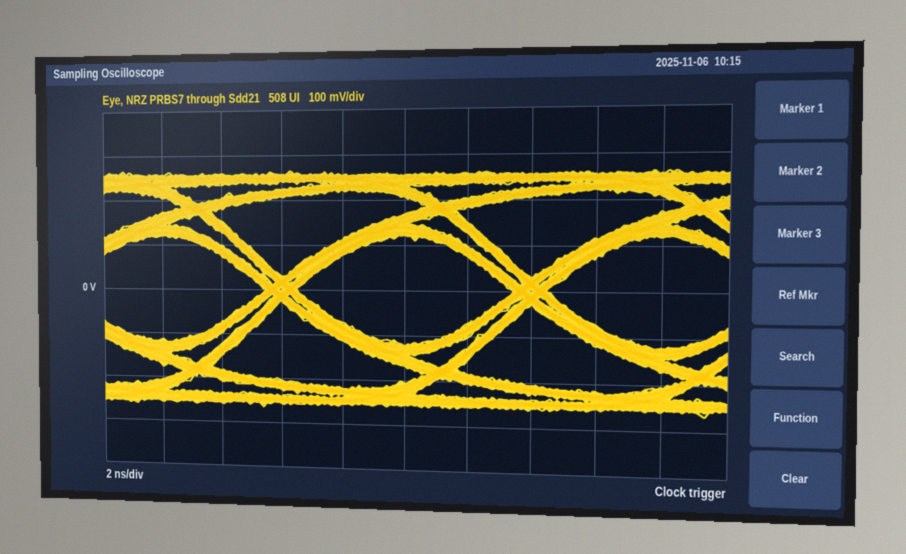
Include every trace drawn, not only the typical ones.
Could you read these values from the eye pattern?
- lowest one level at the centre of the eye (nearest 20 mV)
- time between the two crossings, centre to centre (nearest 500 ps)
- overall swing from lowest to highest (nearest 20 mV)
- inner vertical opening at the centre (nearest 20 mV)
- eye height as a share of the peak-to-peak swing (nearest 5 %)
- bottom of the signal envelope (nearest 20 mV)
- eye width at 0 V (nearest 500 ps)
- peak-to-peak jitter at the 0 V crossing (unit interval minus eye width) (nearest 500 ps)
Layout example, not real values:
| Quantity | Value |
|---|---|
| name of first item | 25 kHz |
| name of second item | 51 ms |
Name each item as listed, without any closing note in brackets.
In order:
| Quantity | Value |
|---|---|
| lowest one level at the centre of the eye | 120 mV |
| time between the two crossings, centre to centre | 8.0 ns |
| overall swing from lowest to highest | 540 mV |
| inner vertical opening at the centre | 240 mV |
| eye height as a share of the peak-to-peak swing | 45 % |
| bottom of the signal envelope | -260 mV |
| eye width at 0 V | 7.0 ns |
| peak-to-peak jitter at the 0 V crossing (unit interval minus eye width) | 1.0 ns |
